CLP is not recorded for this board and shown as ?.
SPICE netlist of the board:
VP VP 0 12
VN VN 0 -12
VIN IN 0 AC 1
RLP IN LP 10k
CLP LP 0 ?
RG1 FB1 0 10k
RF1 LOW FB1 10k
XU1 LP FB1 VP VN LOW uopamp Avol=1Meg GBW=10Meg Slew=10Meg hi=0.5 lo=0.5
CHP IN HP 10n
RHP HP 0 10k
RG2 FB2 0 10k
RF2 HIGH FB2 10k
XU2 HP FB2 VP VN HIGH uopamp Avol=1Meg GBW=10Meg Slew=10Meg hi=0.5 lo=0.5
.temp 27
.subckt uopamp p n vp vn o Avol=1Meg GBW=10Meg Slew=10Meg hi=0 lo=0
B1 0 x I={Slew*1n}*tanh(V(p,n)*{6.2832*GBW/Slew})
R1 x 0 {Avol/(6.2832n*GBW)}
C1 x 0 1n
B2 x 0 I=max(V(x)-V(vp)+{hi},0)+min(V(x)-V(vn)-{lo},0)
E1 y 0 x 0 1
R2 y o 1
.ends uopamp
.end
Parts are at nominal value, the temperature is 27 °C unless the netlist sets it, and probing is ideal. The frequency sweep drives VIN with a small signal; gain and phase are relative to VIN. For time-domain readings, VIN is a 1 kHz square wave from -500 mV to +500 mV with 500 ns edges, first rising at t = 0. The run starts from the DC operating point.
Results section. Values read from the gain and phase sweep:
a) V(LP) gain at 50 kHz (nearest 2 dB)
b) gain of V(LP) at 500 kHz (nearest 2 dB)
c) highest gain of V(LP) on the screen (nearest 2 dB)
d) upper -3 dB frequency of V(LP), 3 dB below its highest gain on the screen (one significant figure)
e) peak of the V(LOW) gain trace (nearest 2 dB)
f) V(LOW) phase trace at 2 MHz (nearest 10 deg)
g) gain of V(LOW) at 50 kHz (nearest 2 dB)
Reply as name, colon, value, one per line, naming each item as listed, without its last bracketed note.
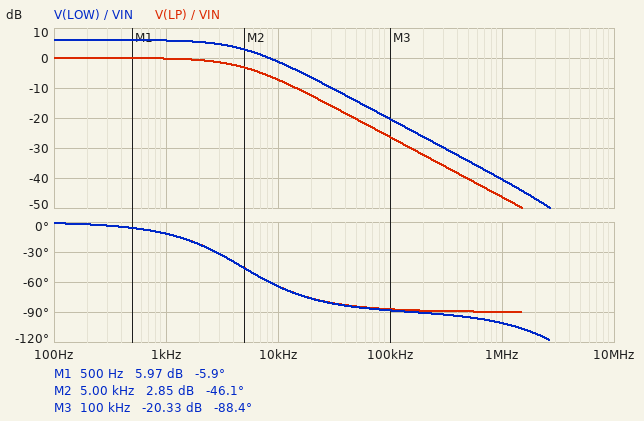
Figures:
V(LP) gain at 50 kHz: -20 dB
gain of V(LP) at 500 kHz: -40 dB
highest gain of V(LP) on the screen: 0 dB
upper -3 dB frequency of V(LP), 3 dB below its highest gain on the screen: 5 kHz
peak of the V(LOW) gain trace: 6 dB
V(LOW) phase trace at 2 MHz: -110 deg
gain of V(LOW) at 50 kHz: -14 dB
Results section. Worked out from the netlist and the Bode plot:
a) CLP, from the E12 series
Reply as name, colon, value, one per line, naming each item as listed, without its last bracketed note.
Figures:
CLP, from the E12 series: 3.3 nF
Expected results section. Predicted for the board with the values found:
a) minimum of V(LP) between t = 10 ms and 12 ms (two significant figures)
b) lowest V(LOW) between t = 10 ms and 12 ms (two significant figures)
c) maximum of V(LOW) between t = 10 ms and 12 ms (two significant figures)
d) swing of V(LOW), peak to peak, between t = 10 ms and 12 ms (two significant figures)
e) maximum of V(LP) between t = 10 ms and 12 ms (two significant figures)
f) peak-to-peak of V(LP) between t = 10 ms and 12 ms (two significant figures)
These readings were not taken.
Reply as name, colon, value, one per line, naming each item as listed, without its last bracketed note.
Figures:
minimum of V(LP) between t = 10 ms and 12 ms: -500 mV
lowest V(LOW) between t = 10 ms and 12 ms: -1.0 V
maximum of V(LOW) between t = 10 ms and 12 ms: 1.0 V
swing of V(LOW), peak to peak, between t = 10 ms and 12 ms: 2.0 V
maximum of V(LP) between t = 10 ms and 12 ms: 500 mV
peak-to-peak of V(LP) between t = 10 ms and 12 ms: 1.0 V
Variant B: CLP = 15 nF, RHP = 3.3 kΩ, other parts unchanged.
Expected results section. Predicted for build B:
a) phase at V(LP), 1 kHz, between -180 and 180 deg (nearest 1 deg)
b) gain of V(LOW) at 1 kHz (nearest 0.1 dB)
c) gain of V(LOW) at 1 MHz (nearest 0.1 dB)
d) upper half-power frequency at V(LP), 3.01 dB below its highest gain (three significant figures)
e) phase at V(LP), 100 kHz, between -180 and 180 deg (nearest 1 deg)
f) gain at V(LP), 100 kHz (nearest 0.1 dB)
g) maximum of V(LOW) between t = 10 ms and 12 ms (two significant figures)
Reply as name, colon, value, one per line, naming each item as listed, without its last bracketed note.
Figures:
phase at V(LP), 1 kHz, between -180 and 180 deg: -43 deg
gain of V(LOW) at 1 kHz: 3.3 dB
gain of V(LOW) at 1 MHz: -53.6 dB
upper half-power frequency at V(LP), 3.01 dB below its highest gain: 1.06 kHz
phase at V(LP), 100 kHz, between -180 and 180 deg: -89 deg
gain at V(LP), 100 kHz: -39.5 dB
maximum of V(LOW) between t = 10 ms and 12 ms: 930 mV
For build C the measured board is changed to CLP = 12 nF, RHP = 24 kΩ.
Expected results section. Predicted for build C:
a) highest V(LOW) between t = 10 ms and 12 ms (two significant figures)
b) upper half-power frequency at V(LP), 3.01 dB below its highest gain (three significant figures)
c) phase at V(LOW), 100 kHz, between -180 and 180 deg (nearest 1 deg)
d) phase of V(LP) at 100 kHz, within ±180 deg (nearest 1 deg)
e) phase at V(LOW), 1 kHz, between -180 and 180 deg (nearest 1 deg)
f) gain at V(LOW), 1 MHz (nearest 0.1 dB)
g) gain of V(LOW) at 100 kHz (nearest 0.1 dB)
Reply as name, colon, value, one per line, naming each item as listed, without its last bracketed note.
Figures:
highest V(LOW) between t = 10 ms and 12 ms: 970 mV
upper half-power frequency at V(LP), 3.01 dB below its highest gain: 1.33 kHz
phase at V(LOW), 100 kHz, between -180 and 180 deg: -90 deg
phase of V(LP) at 100 kHz, within ±180 deg: -89 deg
phase at V(LOW), 1 kHz, between -180 and 180 deg: -37 deg
gain at V(LOW), 1 MHz: -51.7 dB
gain of V(LOW) at 100 kHz: -31.5 dB
